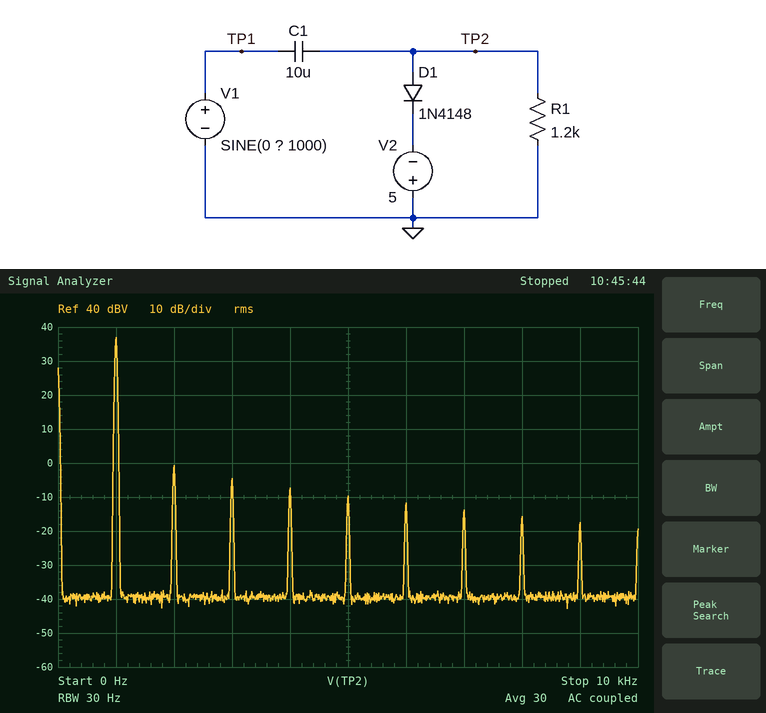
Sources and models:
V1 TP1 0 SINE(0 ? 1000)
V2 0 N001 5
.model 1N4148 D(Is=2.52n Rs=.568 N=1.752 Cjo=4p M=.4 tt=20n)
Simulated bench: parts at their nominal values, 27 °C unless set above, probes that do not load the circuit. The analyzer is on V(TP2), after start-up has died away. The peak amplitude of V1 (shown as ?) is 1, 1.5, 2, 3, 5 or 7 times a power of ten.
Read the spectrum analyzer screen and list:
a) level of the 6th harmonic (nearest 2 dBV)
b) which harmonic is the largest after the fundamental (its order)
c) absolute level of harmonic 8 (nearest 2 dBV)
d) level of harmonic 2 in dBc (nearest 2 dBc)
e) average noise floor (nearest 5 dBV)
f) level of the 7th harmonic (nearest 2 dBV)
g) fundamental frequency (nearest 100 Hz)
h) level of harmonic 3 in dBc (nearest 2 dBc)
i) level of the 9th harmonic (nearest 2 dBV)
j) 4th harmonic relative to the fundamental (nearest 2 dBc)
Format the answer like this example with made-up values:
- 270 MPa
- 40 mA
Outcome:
- -12 dBV
- 2
- -16 dBV
- -38 dBc
- -40 dBV
- -14 dBV
- 1.0 kHz
- -42 dBc
- -18 dBV
- -44 dBc
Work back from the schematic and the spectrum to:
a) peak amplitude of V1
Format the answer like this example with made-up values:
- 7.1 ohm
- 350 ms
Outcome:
- 100 V
